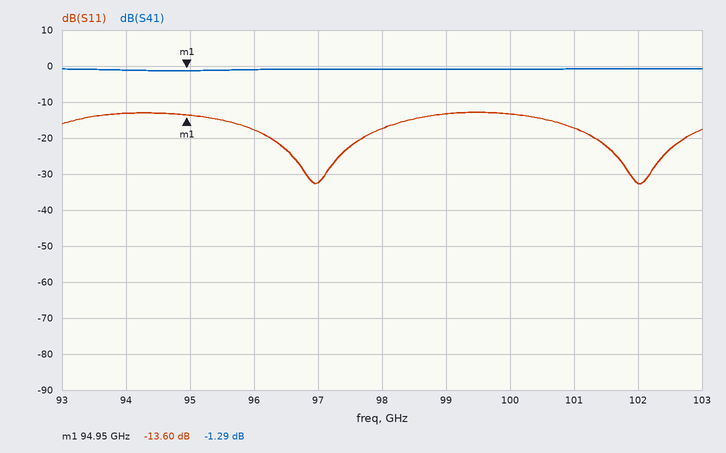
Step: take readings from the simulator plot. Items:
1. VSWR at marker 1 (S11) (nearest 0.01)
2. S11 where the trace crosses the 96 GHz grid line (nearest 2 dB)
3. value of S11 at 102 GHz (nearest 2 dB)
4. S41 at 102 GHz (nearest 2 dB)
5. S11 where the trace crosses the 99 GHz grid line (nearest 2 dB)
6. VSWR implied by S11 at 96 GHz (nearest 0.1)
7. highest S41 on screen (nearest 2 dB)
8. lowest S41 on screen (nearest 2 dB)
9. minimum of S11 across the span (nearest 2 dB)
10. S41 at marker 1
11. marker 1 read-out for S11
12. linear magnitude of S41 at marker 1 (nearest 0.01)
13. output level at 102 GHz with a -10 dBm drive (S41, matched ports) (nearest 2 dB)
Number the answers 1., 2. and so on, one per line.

1. 1.53
2. -18 dB
3. -32 dB
4. 0 dB
5. -14 dB
6. 1.3
7. 0 dB
8. -2 dB
9. -32 dB
10. -1.29 dB
11. -13.60 dB
12. 0.86
13. -10 dBm
